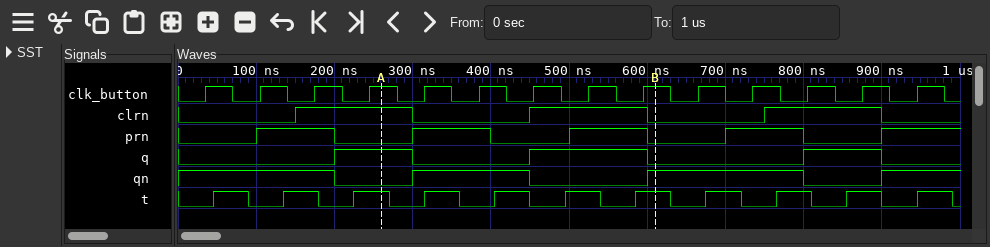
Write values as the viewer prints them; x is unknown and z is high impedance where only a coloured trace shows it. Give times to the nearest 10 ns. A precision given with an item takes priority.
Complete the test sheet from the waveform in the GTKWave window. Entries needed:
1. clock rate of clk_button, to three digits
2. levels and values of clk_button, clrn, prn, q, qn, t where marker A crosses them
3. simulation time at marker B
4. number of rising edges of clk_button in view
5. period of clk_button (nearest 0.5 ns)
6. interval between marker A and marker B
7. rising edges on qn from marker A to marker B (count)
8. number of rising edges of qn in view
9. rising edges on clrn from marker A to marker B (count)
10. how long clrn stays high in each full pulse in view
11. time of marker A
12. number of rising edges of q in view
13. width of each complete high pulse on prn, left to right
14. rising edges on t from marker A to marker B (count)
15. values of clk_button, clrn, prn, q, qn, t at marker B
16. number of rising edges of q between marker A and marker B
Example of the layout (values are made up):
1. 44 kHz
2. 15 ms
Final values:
1. 14.3 MHz
2. clk_button=1, clrn=1, prn=0, q=1, qn=0, t=1
3. 610 ns
4. 14
5. 70 ns
6. 350 ns
7. 2
8. 3
9. 1
10. 150 ns, 150 ns, 150 ns
11. 260 ns
12. 3
13. 100 ns, 100 ns, 100 ns, 100 ns
14. 4
15. clk_button=1, clrn=0, prn=0, q=0, qn=1, t=1
16. 1
